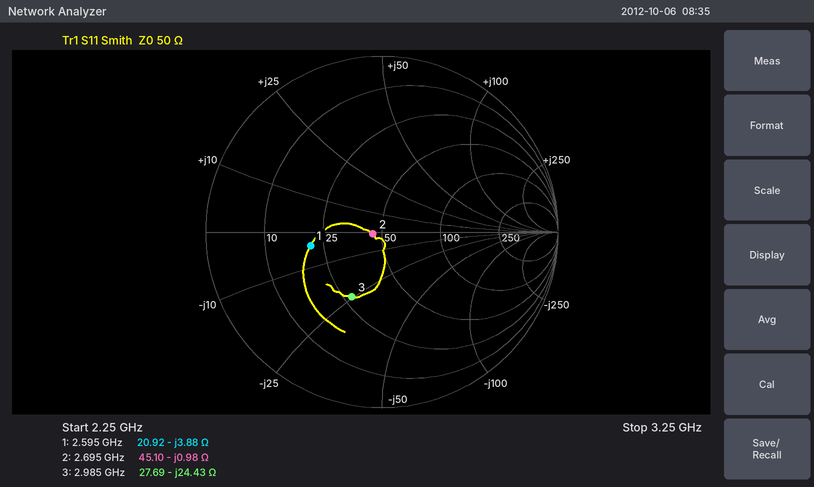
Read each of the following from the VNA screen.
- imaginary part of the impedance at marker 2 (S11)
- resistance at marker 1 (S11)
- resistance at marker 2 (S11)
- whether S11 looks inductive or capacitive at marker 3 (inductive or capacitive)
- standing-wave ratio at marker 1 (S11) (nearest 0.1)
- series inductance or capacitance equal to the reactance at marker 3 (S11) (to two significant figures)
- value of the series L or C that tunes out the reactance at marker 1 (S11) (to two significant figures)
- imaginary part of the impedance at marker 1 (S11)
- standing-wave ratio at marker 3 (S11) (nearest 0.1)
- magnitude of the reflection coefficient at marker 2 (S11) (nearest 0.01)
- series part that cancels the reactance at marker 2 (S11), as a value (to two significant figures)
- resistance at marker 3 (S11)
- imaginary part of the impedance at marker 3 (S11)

-0.98 Ω
20.92 Ω
45.10 Ω
capacitive
2.4
2.2 pF
240 pH
-3.88 Ω
2.4
0.05
58 pH
27.69 Ω
-24.43 Ω
